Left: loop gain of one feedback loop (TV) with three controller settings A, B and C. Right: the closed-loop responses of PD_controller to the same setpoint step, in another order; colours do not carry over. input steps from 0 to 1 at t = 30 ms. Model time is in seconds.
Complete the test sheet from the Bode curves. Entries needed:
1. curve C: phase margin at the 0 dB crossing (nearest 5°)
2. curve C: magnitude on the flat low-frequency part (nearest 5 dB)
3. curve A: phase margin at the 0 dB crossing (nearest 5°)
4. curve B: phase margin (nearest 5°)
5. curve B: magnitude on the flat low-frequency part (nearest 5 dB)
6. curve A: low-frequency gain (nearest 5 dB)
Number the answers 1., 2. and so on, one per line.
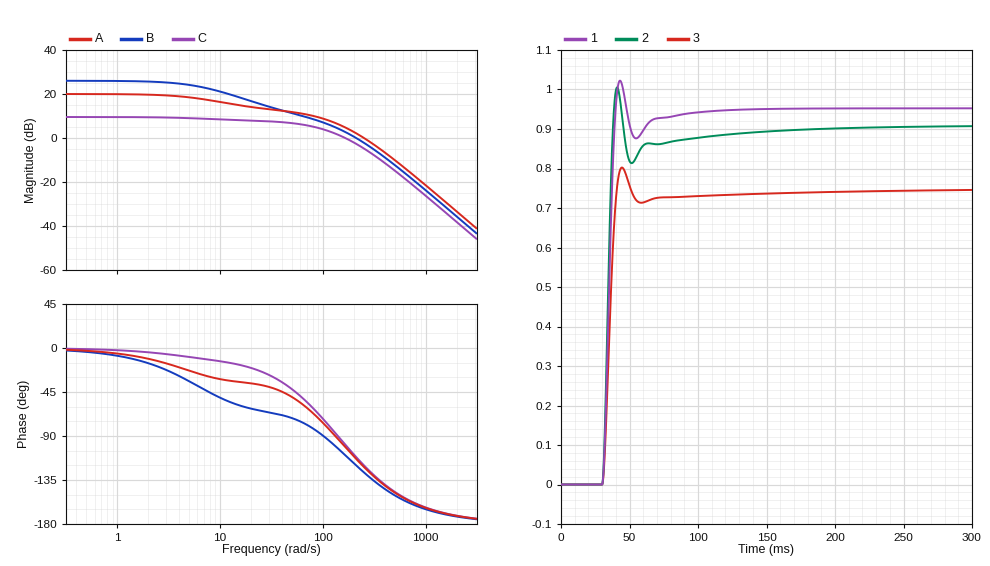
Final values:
1. 80°
2. 10 dB
3. 60°
4. 60°
5. 25 dB
6. 20 dB
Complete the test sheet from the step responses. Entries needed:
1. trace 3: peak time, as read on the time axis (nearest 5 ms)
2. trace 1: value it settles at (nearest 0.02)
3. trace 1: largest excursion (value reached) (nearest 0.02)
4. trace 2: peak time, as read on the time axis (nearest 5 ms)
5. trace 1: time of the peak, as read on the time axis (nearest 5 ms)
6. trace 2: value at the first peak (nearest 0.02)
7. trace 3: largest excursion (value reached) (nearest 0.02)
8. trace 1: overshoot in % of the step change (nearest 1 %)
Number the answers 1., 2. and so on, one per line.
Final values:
1. 45 ms
2. 0.96
3. 1.02
4. 40 ms
5. 45 ms
6. 1.00
7. 0.80
8. 7 %
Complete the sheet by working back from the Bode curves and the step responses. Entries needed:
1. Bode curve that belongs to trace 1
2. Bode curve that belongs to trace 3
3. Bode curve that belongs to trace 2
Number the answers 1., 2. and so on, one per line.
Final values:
1. B
2. C
3. A
